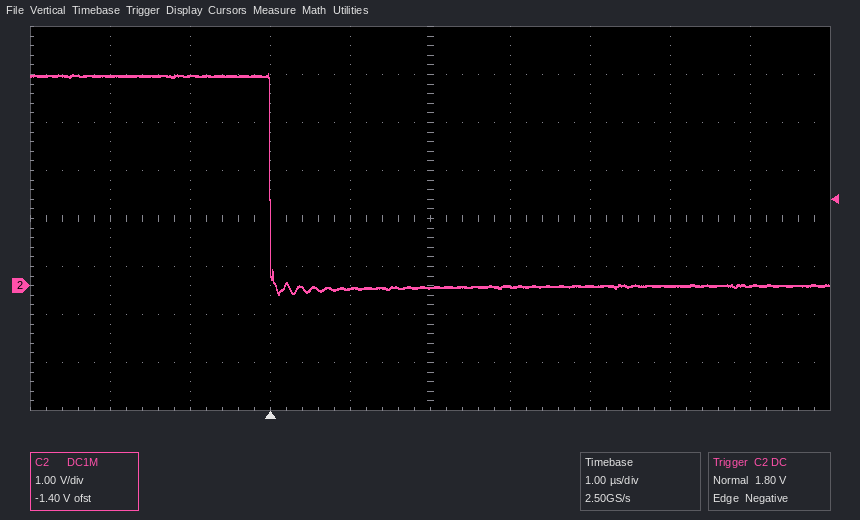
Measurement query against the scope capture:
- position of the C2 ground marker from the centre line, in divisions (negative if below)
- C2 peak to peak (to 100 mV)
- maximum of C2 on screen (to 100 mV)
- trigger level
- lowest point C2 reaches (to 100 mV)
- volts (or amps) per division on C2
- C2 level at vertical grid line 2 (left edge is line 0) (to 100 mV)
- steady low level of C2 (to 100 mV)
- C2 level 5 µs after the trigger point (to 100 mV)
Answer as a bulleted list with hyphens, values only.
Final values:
- -1.4 div
- 4.6 V
- 4.4 V
- 1.80 V
- -200 mV
- 1 V
- 4.4 V
- 0.0 V
- 0.0 V
